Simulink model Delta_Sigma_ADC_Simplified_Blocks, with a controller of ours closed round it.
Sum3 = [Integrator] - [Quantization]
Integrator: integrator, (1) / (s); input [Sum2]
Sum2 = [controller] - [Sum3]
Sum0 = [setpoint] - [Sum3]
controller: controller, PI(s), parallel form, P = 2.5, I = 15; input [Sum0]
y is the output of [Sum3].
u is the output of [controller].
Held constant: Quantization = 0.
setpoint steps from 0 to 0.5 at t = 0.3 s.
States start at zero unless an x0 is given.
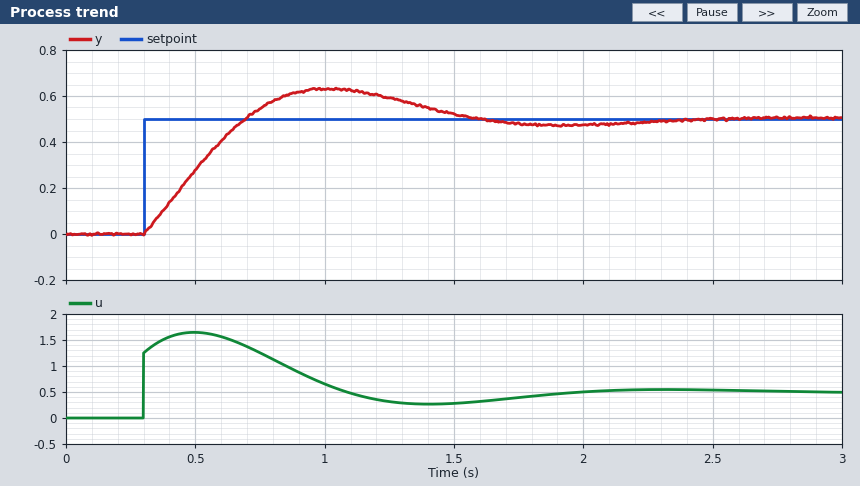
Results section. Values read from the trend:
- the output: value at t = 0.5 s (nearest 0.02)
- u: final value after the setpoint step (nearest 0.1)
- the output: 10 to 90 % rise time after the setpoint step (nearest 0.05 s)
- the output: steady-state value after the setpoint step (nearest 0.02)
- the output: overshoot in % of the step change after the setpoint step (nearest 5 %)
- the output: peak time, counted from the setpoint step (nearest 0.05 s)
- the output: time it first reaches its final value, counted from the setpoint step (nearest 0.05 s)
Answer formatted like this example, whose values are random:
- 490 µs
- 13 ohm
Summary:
- 0.28
- 0.5
- 0.30 s
- 0.50
- 25 %
- 0.70 s
- 0.40 s
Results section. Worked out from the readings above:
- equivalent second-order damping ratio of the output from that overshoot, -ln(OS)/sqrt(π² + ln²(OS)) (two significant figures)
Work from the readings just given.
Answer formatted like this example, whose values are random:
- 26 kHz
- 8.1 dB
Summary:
- 0.40
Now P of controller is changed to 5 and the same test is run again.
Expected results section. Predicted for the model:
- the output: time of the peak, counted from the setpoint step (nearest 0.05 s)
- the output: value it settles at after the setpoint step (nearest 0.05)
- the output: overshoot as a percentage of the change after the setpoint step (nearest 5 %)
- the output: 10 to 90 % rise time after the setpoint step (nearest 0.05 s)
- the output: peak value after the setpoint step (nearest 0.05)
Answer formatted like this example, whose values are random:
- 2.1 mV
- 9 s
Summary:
- 0.65 s
- 0.50
- 10 %
- 0.25 s
- 0.55
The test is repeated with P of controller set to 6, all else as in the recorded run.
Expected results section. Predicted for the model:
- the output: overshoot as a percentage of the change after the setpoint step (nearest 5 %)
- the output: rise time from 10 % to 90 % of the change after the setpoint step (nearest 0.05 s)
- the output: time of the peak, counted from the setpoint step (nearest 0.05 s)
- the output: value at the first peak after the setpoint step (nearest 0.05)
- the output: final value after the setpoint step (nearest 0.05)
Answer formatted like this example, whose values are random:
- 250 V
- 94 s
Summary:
- 10 %
- 0.25 s
- 0.60 s
- 0.55
- 0.50
